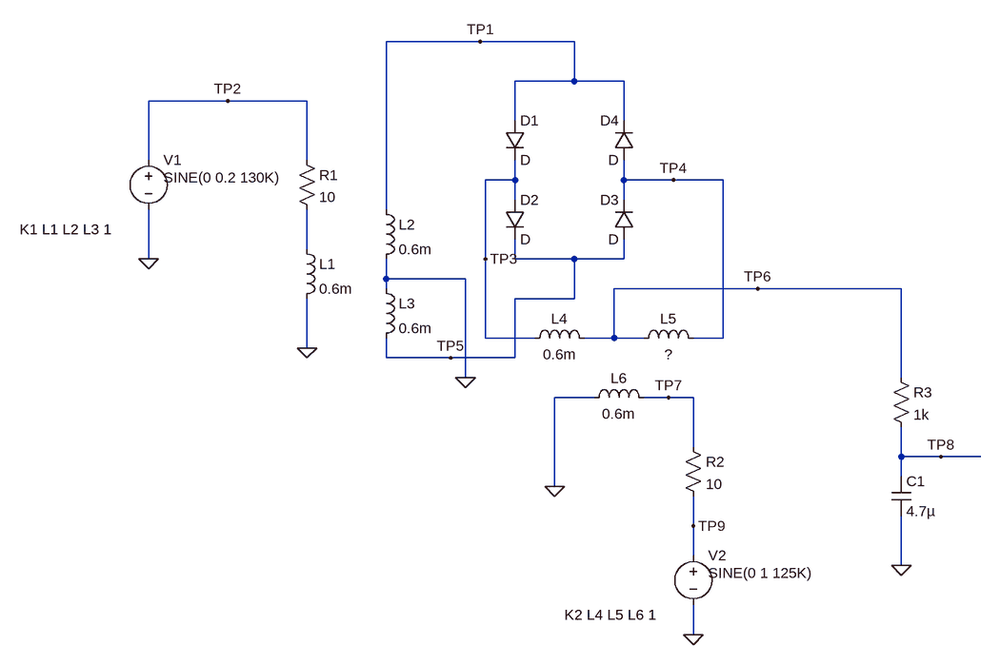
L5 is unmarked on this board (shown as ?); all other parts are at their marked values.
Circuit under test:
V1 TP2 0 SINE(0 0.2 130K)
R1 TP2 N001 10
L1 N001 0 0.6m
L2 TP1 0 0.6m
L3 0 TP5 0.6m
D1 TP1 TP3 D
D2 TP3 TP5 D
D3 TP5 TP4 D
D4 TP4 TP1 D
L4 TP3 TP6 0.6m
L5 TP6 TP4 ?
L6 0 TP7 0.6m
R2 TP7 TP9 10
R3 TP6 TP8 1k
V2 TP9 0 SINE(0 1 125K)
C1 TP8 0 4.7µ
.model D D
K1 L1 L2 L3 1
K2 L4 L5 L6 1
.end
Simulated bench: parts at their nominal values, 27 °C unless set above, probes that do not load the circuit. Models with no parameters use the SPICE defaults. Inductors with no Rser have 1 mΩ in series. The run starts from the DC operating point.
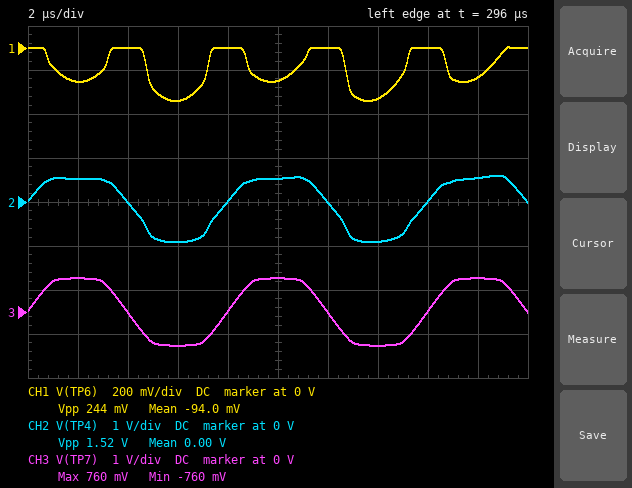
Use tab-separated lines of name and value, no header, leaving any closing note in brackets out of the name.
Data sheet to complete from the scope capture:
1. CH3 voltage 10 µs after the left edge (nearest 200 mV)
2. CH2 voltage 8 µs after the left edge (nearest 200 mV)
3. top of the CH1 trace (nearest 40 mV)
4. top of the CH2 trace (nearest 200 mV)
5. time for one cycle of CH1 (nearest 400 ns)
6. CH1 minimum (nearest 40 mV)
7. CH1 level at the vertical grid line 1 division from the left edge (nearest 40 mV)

CH3 voltage 10 µs after the left edge	800 mV
CH2 voltage 8 µs after the left edge	0 V
top of the CH1 trace	0 V
top of the CH2 trace	600 mV
time for one cycle of CH1	8.0 µs
CH1 minimum	-240 mV
CH1 level at the vertical grid line 1 division from the left edge	-160 mV
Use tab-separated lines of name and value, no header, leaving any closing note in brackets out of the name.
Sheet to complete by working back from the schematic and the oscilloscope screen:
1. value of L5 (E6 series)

value of L5	470 µH
